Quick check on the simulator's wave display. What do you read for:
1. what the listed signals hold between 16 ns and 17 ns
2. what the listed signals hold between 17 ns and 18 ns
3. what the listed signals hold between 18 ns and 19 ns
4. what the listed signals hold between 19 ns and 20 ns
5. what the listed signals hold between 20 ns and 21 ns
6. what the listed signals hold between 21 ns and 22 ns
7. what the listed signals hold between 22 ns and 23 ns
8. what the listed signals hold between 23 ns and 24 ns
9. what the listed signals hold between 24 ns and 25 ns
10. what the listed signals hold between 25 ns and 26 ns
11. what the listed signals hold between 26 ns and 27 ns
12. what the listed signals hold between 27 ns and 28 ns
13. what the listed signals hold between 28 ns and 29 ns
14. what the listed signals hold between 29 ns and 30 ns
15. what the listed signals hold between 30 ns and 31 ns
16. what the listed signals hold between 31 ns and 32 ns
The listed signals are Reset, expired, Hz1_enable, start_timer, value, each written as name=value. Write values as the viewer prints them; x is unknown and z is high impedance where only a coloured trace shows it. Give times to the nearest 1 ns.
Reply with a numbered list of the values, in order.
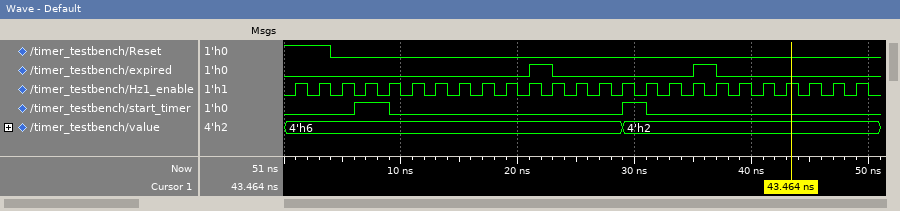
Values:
1. Reset=0, expired=0, Hz1_enable=0, start_timer=0, value=4'h6
2. Reset=0, expired=0, Hz1_enable=1, start_timer=0, value=4'h6
3. Reset=0, expired=0, Hz1_enable=0, start_timer=0, value=4'h6
4. Reset=0, expired=0, Hz1_enable=1, start_timer=0, value=4'h6
5. Reset=0, expired=0, Hz1_enable=0, start_timer=0, value=4'h6
6. Reset=0, expired=1, Hz1_enable=1, start_timer=0, value=4'h6
7. Reset=0, expired=1, Hz1_enable=0, start_timer=0, value=4'h6
8. Reset=0, expired=0, Hz1_enable=1, start_timer=0, value=4'h6
9. Reset=0, expired=0, Hz1_enable=0, start_timer=0, value=4'h6
10. Reset=0, expired=0, Hz1_enable=1, start_timer=0, value=4'h6
11. Reset=0, expired=0, Hz1_enable=0, start_timer=0, value=4'h6
12. Reset=0, expired=0, Hz1_enable=1, start_timer=0, value=4'h6
13. Reset=0, expired=0, Hz1_enable=0, start_timer=0, value=4'h6
14. Reset=0, expired=0, Hz1_enable=1, start_timer=1, value=4'h2
15. Reset=0, expired=0, Hz1_enable=0, start_timer=1, value=4'h2
16. Reset=0, expired=0, Hz1_enable=1, start_timer=0, value=4'h2
